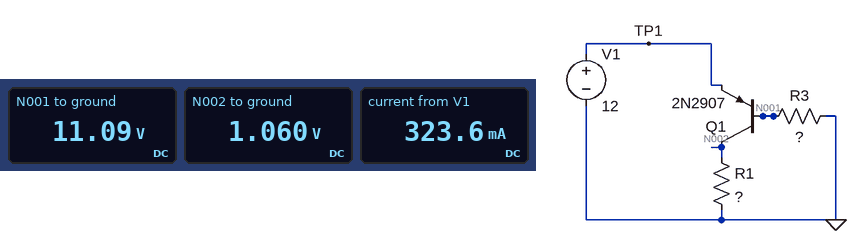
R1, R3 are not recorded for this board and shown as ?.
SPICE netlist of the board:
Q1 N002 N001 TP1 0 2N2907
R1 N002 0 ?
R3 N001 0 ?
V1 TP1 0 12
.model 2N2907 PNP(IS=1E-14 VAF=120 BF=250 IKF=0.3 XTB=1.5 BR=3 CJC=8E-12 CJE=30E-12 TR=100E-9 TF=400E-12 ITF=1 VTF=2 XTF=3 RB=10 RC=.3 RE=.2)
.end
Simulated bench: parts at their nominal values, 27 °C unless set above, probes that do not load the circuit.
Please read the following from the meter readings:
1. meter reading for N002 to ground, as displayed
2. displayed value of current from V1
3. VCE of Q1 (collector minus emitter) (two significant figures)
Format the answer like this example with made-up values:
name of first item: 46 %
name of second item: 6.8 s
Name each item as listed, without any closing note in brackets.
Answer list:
meter reading for N002 to ground, as displayed: 1.060 V
displayed value of current from V1: 323.6 mA
VCE of Q1 (collector minus emitter): -11 V
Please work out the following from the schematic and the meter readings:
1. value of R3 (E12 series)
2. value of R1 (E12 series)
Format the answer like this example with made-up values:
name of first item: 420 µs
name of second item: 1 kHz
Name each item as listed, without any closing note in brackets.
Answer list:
value of R3: 4.7 kΩ
value of R1: 3.3 Ω
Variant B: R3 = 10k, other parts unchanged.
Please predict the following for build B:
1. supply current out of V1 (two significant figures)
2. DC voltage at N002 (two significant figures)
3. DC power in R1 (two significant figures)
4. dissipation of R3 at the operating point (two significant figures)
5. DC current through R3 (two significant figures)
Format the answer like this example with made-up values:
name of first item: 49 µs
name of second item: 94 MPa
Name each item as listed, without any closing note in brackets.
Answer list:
supply current out of V1: 190 mA
DC voltage at N002: 630 mV
DC power in R1: 120 mW
dissipation of R3 at the operating point: 12 mW
DC current through R3: 1.1 mA
